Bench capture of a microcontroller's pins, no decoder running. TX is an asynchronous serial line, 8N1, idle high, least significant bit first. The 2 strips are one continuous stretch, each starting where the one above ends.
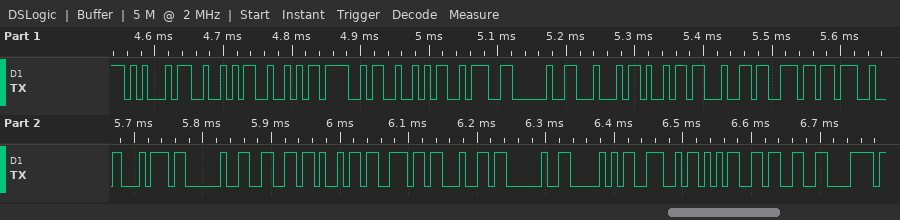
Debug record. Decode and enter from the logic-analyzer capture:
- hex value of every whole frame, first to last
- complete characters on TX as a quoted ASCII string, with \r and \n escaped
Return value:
45 52 52 4F 52 3A 20 44 69 64 6E 27 74 20 66 69 6E 64 20 50 4E 35 33 78
"ERROR: Didn't find PN53x"
